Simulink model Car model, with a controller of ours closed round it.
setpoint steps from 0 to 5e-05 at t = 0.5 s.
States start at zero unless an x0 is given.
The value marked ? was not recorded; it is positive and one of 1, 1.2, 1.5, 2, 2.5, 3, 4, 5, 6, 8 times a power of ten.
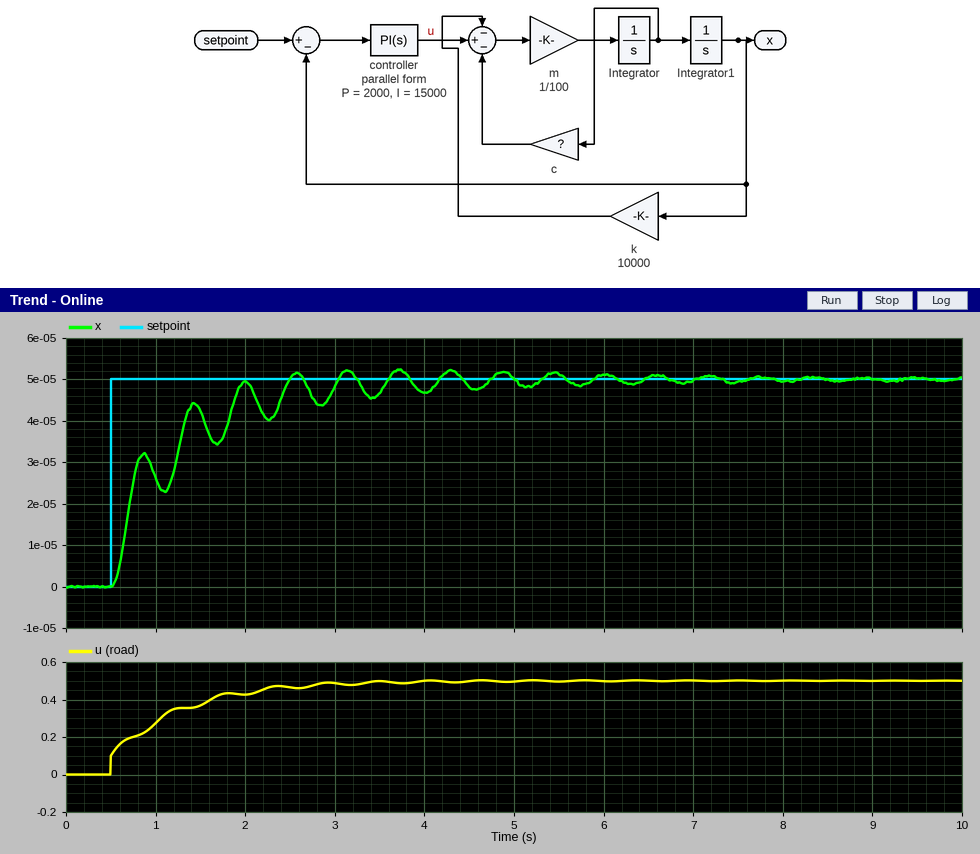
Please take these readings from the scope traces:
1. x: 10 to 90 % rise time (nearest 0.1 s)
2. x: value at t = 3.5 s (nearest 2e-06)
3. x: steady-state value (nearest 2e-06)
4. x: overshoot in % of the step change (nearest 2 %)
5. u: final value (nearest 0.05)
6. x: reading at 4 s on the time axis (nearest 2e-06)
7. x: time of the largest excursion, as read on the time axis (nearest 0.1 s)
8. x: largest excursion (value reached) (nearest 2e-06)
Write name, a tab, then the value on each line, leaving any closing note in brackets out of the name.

x: 10 to 90 % rise time	1.3 s
x: value at t = 3.5 s	0.000046
x: steady-state value	0.000050
x: overshoot in % of the step change	4 %
u: final value	0.50
x: reading at 4 s on the time axis	0.000046
x: time of the largest excursion, as read on the time axis	3.7 s
x: largest excursion (value reached)	0.000052
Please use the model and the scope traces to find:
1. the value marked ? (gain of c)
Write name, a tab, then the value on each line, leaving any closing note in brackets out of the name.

the value marked ?	200
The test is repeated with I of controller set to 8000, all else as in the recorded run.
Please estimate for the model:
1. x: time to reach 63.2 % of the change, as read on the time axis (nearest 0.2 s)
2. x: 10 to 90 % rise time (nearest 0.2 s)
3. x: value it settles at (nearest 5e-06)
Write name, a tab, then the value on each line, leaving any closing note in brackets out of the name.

x: time to reach 63.2 % of the change, as read on the time axis	1.4 s
x: 10 to 90 % rise time	3.0 s
x: value it settles at	0.000050
